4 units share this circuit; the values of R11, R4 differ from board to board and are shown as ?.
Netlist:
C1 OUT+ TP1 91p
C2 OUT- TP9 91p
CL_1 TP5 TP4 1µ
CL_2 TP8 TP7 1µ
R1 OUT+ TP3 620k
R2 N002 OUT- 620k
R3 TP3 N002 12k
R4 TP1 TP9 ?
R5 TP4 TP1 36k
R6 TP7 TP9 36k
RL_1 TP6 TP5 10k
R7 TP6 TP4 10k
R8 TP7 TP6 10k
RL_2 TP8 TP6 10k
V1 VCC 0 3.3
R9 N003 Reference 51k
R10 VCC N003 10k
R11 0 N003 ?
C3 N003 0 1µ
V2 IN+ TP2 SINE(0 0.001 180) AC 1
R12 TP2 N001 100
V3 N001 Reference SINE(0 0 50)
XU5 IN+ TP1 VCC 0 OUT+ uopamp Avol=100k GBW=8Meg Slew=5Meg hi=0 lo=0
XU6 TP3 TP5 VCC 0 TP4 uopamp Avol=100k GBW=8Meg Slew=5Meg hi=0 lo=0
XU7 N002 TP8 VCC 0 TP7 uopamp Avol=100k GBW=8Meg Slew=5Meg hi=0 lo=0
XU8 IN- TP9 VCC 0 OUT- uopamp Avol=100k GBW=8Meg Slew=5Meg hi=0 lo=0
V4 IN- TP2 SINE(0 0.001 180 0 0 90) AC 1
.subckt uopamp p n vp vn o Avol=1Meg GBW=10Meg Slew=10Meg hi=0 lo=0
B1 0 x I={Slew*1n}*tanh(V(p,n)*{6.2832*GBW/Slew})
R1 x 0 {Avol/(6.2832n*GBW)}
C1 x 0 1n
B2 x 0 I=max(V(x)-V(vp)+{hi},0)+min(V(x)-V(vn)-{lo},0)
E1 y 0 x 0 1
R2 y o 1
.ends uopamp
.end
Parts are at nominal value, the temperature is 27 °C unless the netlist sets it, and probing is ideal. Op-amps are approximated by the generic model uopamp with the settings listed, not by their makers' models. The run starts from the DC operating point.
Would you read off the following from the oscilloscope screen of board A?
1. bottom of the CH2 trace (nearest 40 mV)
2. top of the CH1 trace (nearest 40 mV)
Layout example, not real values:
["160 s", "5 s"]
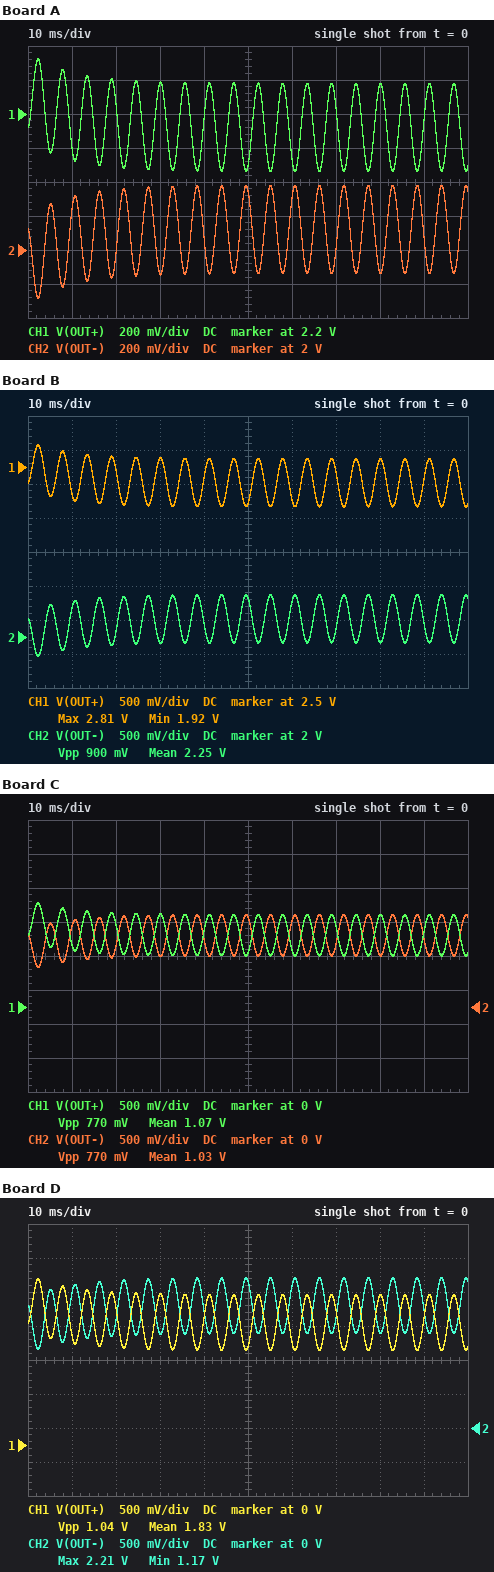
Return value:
["1.72 V", "2.52 V"]
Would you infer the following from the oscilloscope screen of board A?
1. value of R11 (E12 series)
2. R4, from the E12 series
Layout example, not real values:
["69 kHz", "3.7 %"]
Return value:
["18 kΩ", "27 kΩ"]
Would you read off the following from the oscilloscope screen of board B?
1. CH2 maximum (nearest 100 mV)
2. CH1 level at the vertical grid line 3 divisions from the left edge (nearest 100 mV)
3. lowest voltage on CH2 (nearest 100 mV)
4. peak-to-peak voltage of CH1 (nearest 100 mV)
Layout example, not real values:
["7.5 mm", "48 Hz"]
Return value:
["2.6 V", "2.6 V", "1.7 V", "900 mV"]
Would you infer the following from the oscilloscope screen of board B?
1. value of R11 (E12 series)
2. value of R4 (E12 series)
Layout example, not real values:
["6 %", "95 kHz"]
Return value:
["22 kΩ", "18 kΩ"]
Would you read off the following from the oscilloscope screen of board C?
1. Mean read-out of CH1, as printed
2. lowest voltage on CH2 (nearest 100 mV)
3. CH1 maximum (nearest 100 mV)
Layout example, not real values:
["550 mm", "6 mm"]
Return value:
["1.07 V", "600 mV", "1.5 V"]
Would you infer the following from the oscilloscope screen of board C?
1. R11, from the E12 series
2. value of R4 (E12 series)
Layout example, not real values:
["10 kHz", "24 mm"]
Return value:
["4.7 kΩ", "22 kΩ"]
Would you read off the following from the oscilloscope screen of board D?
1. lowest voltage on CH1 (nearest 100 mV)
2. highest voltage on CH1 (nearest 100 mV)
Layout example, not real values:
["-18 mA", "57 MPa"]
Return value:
["1.4 V", "2.4 V"]
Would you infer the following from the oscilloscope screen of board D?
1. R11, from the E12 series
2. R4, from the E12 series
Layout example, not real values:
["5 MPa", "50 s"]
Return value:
["12 kΩ", "15 kΩ"]
